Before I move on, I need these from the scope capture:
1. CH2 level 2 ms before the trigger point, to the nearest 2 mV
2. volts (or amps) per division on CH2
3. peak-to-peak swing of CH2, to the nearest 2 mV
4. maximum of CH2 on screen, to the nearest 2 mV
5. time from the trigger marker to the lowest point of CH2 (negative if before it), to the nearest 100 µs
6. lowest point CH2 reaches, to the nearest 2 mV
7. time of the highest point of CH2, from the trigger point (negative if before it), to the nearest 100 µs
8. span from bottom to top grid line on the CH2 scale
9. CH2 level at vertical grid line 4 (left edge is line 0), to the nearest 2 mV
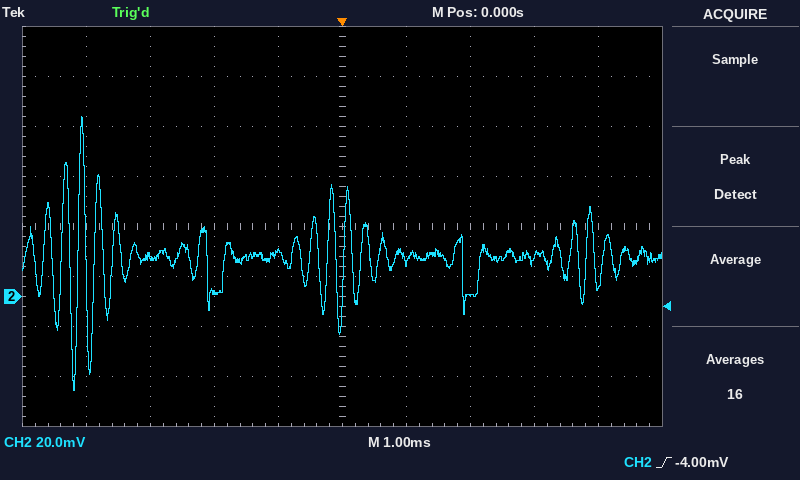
2 mV
20 mV
110 mV
72 mV
-4.2 ms
-38 mV
-4.1 ms
160 mV
18 mV
